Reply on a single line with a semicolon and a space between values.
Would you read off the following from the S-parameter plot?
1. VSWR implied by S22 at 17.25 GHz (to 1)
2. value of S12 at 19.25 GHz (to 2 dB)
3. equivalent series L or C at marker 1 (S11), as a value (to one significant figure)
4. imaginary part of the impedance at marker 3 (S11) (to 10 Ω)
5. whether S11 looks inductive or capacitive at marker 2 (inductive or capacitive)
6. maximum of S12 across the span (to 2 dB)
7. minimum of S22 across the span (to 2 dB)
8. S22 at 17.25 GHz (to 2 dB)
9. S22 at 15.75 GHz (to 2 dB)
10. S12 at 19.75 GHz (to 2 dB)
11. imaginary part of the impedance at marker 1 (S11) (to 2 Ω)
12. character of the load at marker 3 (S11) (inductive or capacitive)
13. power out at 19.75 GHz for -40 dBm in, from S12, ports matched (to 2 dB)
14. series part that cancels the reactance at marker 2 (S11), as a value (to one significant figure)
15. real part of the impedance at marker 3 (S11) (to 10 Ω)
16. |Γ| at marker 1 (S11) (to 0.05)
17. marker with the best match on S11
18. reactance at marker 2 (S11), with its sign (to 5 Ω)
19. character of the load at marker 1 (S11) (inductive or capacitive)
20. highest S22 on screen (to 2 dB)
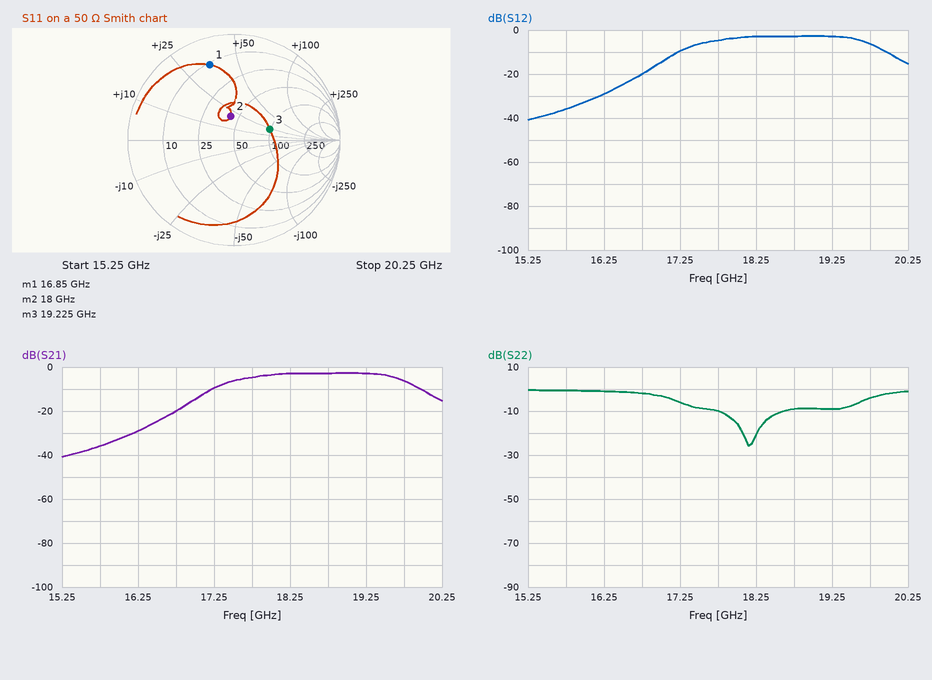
3; -2 dB; 300 pH; +20 Ω; inductive; -2 dB; -26 dB; -6 dB; 0 dB; -6 dB; +36 Ω; inductive; -46 dBm; 400 fF; 100 Ω; 0.75; marker 2; +20 Ω; inductive; 0 dB
